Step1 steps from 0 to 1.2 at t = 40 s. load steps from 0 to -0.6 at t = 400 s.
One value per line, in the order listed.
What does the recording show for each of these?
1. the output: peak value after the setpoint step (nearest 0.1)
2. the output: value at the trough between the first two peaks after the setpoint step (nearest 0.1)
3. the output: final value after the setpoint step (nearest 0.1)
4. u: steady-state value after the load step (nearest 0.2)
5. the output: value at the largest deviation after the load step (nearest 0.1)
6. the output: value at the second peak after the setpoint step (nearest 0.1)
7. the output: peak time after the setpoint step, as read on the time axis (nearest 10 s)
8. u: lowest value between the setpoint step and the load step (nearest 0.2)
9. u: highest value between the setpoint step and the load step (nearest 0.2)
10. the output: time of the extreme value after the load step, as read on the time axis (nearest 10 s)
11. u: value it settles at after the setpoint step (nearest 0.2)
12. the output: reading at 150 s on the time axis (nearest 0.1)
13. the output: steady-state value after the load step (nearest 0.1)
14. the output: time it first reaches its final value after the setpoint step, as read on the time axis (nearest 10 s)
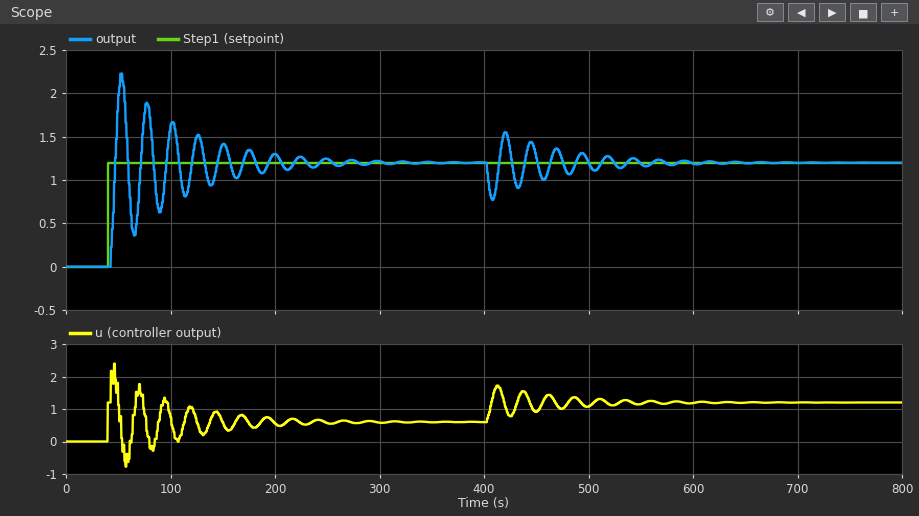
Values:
2.2
0.4
1.2
1.2
0.8
1.9
50 s
-0.8
2.4
410 s
0.6
1.4
1.2
50 s
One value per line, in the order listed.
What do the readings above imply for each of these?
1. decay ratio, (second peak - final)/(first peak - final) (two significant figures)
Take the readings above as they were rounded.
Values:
0.70
